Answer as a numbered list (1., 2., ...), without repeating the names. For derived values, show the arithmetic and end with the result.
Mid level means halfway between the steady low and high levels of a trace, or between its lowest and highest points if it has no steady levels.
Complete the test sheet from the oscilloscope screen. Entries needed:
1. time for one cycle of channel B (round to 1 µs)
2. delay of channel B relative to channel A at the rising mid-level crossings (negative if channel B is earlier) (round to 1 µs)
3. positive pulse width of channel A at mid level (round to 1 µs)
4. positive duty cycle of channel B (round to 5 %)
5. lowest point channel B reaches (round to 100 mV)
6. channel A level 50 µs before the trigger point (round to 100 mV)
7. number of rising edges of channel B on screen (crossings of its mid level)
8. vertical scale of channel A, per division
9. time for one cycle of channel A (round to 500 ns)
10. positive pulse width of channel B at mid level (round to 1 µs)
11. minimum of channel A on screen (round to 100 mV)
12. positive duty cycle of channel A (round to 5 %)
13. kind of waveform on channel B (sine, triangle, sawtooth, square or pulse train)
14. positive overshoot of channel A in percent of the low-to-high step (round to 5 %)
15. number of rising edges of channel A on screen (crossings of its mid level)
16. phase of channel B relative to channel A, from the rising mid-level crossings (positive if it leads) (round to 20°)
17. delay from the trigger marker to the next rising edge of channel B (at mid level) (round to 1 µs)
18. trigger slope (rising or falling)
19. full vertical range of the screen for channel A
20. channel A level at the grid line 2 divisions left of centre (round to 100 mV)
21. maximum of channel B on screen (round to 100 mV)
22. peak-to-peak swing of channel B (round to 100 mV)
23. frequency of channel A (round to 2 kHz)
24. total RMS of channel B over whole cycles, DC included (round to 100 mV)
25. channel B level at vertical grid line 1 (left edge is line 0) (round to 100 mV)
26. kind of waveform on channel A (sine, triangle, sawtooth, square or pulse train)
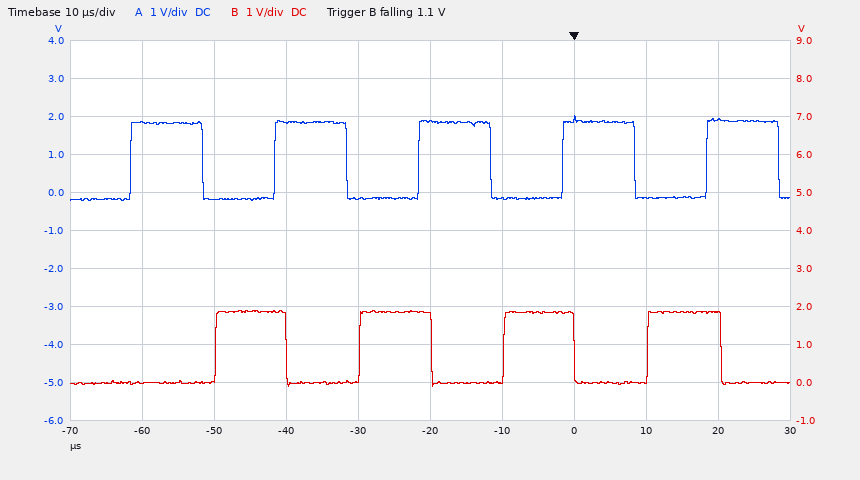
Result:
1. 20 µs
2. -8 µs
3. 10 µs
4. 10 µs / 20 µs ≈ 50 %
5. -100 mV
6. -200 mV
7. 4
8. 1 V
9. 20.0 µs
10. 10 µs
11. -200 mV
12. 10 µs / 20.0 µs ≈ 50 %
13. square
14. 10 %
15. 5
16. −360° × (-8 µs) / 20.0 µs ≈ +144°, so +140° to the nearest 20°
17. 10 µs
18. falling
19. 10 V
20. 1.8 V
21. 1.9 V
22. 1.9 V − (-100 mV) = 2.0 V
23. 1 / 20.0 µs ≈ 50 kHz
24. √(0.5 × (1.9 V)² + 0.5 × (-100 mV)²) ≈ 1.3 V
25. 0.0 V
26. square
